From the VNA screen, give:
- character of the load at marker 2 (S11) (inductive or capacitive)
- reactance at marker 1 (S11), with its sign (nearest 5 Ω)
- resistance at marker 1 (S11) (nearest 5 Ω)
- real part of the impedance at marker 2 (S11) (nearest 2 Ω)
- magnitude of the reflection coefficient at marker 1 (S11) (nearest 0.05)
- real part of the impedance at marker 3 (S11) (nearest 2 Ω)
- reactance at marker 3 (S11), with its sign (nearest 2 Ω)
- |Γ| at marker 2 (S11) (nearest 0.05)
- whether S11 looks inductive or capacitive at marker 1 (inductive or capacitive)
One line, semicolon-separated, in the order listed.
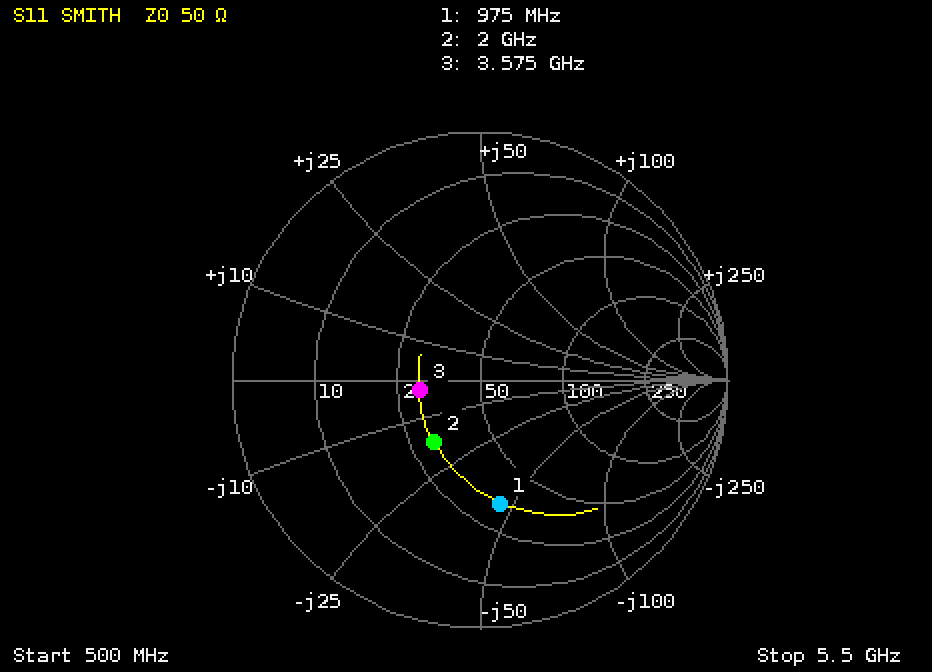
capacitive; -45 Ω; 35 Ω; 30 Ω; 0.50; 30 Ω; -2 Ω; 0.30; capacitive
